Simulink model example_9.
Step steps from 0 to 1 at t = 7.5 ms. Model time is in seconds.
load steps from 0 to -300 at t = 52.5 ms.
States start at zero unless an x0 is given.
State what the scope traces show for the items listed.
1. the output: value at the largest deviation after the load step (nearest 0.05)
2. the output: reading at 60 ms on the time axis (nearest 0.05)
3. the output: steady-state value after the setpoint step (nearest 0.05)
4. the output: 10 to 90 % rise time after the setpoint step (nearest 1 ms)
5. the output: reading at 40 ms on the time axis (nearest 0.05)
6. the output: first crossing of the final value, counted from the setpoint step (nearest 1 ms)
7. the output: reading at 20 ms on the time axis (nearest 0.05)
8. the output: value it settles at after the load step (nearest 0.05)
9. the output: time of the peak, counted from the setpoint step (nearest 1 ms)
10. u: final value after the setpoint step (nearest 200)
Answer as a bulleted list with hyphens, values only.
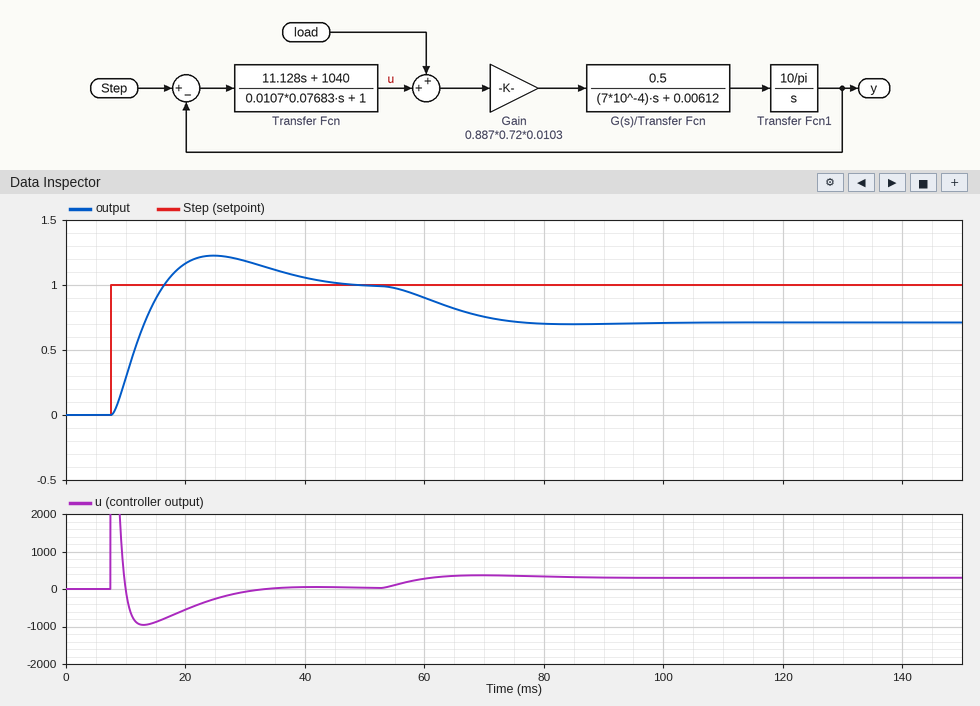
- 0.70
- 0.90
- 1.00
- 6 ms
- 1.05
- 9 ms
- 1.15
- 0.70
- 17 ms
- 0
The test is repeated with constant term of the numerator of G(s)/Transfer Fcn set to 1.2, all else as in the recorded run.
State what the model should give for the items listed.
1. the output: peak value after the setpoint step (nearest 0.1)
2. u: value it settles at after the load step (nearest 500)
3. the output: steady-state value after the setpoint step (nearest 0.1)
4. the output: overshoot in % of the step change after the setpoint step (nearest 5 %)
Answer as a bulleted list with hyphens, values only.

- 1.2
- 500
- 1.0
- 15 %
